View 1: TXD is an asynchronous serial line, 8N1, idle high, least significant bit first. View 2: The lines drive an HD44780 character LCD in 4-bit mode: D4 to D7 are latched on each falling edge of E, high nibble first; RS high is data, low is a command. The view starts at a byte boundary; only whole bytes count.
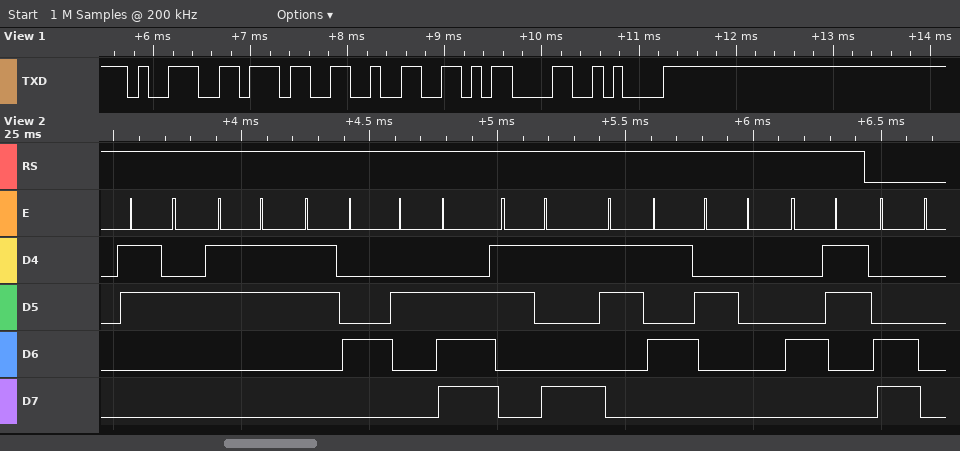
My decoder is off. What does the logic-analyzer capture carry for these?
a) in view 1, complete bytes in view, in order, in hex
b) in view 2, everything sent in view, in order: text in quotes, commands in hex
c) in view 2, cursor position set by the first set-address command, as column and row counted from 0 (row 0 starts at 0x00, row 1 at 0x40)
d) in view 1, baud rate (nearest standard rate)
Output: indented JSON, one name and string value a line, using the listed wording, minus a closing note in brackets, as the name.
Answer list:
{
  "in view 1, complete bytes in view, in order, in hex": "39 37 32 0D 0A",
  "in view 2, everything sent in view, in order: text in quotes, commands in hex": "\"234.95 C\" 0xC0",
  "in view 2, cursor position set by the first set-address command, as column and row counted from 0": "column 0, row 1",
  "in view 1, baud rate": "9600 baud"
}
